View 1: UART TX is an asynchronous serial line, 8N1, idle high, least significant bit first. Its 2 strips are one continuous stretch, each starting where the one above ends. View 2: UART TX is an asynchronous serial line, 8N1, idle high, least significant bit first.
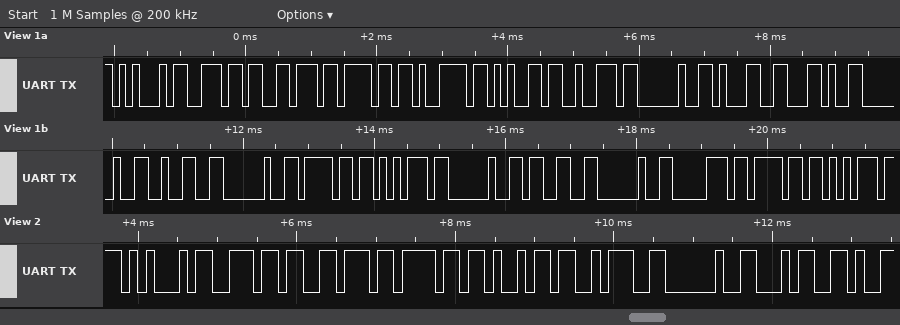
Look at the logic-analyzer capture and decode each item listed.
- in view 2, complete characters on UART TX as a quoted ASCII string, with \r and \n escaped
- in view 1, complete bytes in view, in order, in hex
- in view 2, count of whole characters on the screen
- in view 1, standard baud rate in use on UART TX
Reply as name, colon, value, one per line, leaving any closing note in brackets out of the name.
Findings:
in view 2, complete characters on UART TX as a quoted ASCII string, with \r and \n escaped: "Envoi: 4"
in view 1, complete bytes in view, in order, in hex: 45 6E 76 6F 79 65 72 20 31 2C 20 32 20 6F 75 20 33 20 70 6F 75
in view 2, count of whole characters on the screen: 8
in view 1, standard baud rate in use on UART TX: 9600 baud
